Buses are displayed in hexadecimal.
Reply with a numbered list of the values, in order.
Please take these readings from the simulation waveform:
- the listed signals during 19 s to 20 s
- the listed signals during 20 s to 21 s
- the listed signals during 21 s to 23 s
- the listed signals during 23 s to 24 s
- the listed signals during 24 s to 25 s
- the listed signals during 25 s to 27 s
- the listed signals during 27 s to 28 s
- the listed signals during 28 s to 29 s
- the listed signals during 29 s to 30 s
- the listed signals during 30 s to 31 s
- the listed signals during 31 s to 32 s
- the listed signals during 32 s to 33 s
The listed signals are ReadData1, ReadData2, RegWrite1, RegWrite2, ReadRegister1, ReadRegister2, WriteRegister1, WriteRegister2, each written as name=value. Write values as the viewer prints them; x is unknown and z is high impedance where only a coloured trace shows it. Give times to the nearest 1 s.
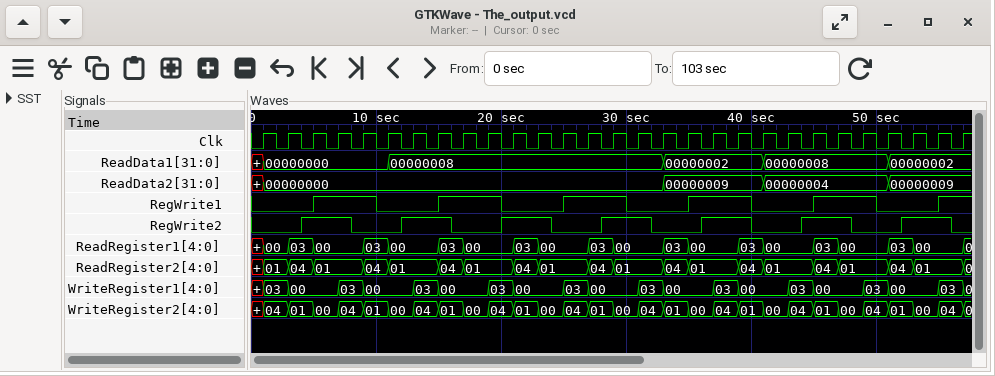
1. ReadData1=00000008, ReadData2=00000000, RegWrite1=1, RegWrite2=0, ReadRegister1=00, ReadRegister2=01, WriteRegister1=03, WriteRegister2=04
2. ReadData1=00000008, ReadData2=00000000, RegWrite1=0, RegWrite2=1, ReadRegister1=00, ReadRegister2=01, WriteRegister1=03, WriteRegister2=04
3. ReadData1=00000008, ReadData2=00000000, RegWrite1=0, RegWrite2=1, ReadRegister1=03, ReadRegister2=04, WriteRegister1=00, WriteRegister2=01
4. ReadData1=00000008, ReadData2=00000000, RegWrite1=0, RegWrite2=1, ReadRegister1=00, ReadRegister2=01, WriteRegister1=00, WriteRegister2=00
5. ReadData1=00000008, ReadData2=00000000, RegWrite1=0, RegWrite2=0, ReadRegister1=00, ReadRegister2=01, WriteRegister1=00, WriteRegister2=00
6. ReadData1=00000008, ReadData2=00000000, RegWrite1=1, RegWrite2=0, ReadRegister1=00, ReadRegister2=01, WriteRegister1=03, WriteRegister2=04
7. ReadData1=00000008, ReadData2=00000000, RegWrite1=1, RegWrite2=0, ReadRegister1=03, ReadRegister2=04, WriteRegister1=00, WriteRegister2=01
8. ReadData1=00000008, ReadData2=00000000, RegWrite1=1, RegWrite2=1, ReadRegister1=03, ReadRegister2=04, WriteRegister1=00, WriteRegister2=01
9. ReadData1=00000008, ReadData2=00000000, RegWrite1=1, RegWrite2=1, ReadRegister1=00, ReadRegister2=01, WriteRegister1=00, WriteRegister2=00
10. ReadData1=00000008, ReadData2=00000000, RegWrite1=0, RegWrite2=1, ReadRegister1=00, ReadRegister2=01, WriteRegister1=00, WriteRegister2=00
11. ReadData1=00000008, ReadData2=00000000, RegWrite1=0, RegWrite2=1, ReadRegister1=00, ReadRegister2=01, WriteRegister1=03, WriteRegister2=04
12. ReadData1=00000008, ReadData2=00000000, RegWrite1=0, RegWrite2=0, ReadRegister1=00, ReadRegister2=01, WriteRegister1=03, WriteRegister2=04
